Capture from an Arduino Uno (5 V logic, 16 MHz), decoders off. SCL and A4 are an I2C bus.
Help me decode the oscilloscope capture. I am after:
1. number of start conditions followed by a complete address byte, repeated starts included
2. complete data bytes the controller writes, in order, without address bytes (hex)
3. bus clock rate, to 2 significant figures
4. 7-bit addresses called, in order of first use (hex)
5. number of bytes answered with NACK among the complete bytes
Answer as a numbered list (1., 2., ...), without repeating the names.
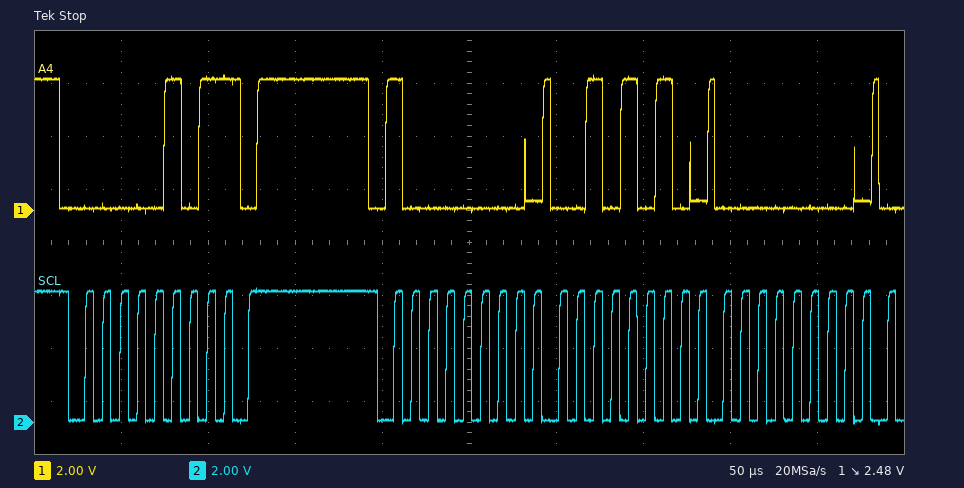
1. 2
2. 2A 00
3. 100 kHz
4. 0x02 0x40
5. 1
